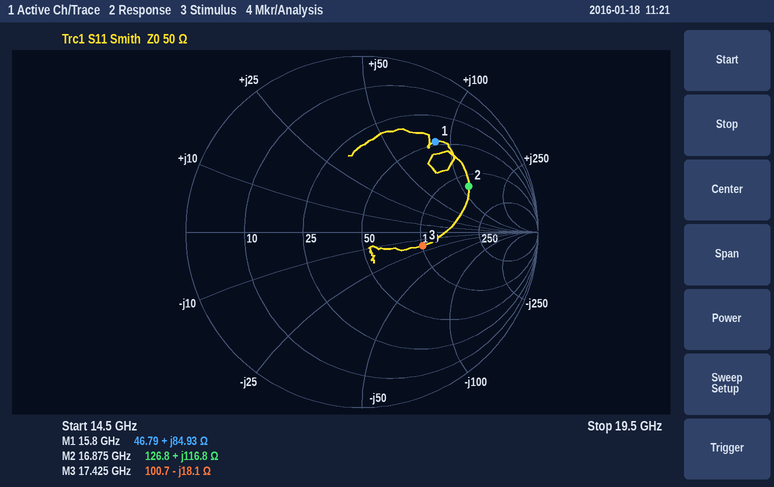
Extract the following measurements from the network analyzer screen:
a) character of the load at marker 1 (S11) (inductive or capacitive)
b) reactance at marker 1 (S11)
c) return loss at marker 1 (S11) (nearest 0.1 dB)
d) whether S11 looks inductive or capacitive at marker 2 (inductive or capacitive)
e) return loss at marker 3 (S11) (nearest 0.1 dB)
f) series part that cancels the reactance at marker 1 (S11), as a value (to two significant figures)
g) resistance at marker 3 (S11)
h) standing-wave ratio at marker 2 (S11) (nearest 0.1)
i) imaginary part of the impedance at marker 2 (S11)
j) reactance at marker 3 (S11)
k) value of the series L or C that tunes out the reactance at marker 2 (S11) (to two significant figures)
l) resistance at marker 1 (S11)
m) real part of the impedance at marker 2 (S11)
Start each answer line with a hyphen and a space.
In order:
- inductive
- +84.93 Ω
- 3.6 dB
- inductive
- 9.0 dB
- 120 fF
- 100.7 Ω
- 4.9
- +116.8 Ω
- -18.1 Ω
- 81 fF
- 46.79 Ω
- 126.8 Ω
